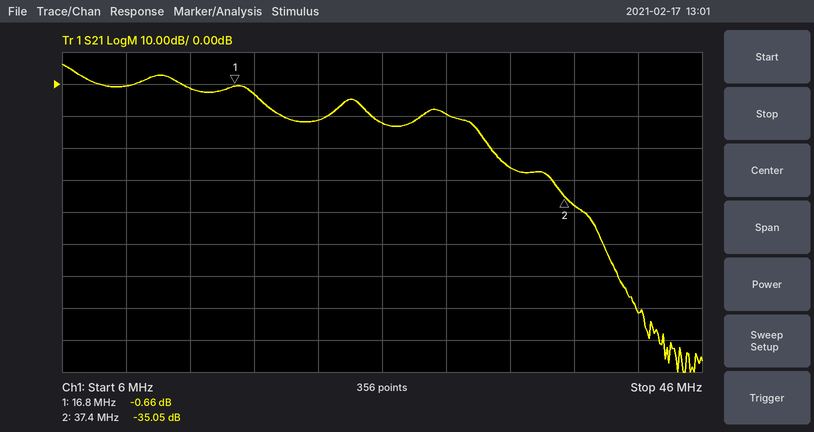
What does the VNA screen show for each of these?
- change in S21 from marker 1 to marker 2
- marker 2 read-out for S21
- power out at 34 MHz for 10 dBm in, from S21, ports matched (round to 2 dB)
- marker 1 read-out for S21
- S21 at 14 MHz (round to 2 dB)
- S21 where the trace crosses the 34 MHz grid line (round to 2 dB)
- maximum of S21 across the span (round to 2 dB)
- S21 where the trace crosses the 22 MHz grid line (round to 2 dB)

-34.39 dB
-35.05 dB
-16 dBm
-0.66 dB
-2 dB
-26 dB
6 dB
-12 dB
